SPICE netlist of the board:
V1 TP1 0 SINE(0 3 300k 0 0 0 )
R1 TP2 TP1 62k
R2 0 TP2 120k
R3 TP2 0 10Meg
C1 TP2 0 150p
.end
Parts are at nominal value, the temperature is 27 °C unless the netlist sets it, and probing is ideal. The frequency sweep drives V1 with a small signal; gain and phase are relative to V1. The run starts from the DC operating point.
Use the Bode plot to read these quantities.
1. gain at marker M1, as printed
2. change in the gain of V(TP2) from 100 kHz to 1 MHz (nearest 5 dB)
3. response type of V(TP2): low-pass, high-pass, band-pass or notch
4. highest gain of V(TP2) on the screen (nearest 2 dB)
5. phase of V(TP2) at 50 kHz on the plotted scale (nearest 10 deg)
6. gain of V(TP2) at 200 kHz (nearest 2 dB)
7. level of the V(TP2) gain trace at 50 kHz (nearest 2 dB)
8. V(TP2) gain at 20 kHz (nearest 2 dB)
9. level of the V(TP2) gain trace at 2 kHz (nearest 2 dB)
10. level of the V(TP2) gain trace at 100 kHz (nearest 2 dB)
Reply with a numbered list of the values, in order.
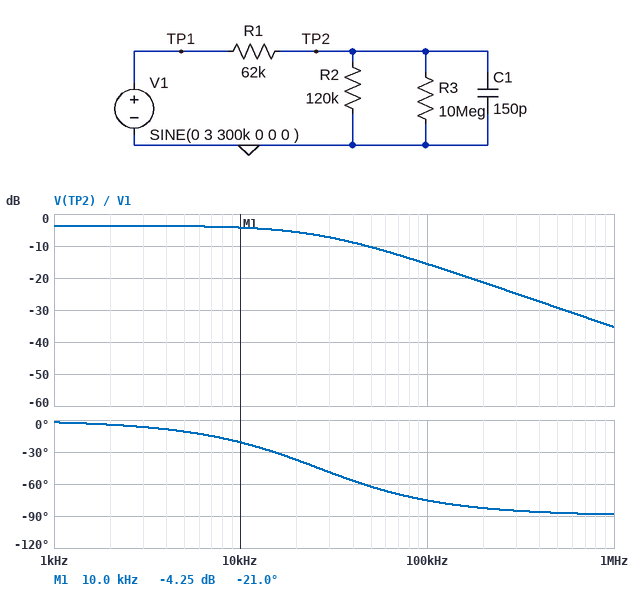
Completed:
1. -4.25 dB
2. -20 dB
3. low-pass
4. -4 dB
5. -60 deg
6. -22 dB
7. -10 dB
8. -6 dB
9. -4 dB
10. -16 dB
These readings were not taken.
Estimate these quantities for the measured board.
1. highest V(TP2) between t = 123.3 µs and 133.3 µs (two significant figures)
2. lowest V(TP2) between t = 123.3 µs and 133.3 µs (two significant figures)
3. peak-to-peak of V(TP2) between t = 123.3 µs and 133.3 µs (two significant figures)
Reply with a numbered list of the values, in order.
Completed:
1. 170 mV
2. -170 mV
3. 340 mV
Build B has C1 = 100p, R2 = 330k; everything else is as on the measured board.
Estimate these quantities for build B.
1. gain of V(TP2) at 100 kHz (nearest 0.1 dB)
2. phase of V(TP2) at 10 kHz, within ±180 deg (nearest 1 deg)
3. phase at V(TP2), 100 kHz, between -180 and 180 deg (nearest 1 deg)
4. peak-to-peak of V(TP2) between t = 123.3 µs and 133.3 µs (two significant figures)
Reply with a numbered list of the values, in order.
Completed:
1. -12.2 dB
2. -18 deg
3. -73 deg
4. 510 mV
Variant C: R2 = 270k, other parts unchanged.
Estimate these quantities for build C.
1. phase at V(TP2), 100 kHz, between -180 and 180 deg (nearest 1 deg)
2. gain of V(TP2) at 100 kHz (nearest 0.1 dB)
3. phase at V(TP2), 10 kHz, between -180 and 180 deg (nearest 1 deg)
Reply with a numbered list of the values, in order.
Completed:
1. -78 deg
2. -15.5 dB
3. -25 deg
